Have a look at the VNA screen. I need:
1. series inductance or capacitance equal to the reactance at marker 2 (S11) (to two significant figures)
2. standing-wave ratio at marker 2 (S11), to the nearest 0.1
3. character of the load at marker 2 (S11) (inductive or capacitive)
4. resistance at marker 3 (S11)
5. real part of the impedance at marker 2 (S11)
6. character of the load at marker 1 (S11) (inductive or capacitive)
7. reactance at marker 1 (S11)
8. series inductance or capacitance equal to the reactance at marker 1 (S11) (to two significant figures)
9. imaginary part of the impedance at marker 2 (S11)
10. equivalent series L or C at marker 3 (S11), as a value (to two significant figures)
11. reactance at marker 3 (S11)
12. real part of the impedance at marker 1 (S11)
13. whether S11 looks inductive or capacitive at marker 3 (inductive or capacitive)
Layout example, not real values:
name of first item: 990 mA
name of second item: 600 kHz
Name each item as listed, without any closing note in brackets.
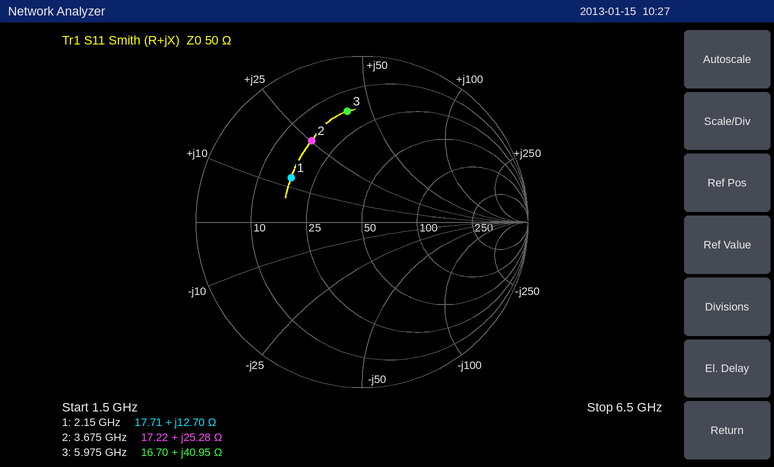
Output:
series inductance or capacitance equal to the reactance at marker 2 (S11): 1.1 nH
standing-wave ratio at marker 2 (S11), to the nearest 0.1: 3.7
character of the load at marker 2 (S11): inductive
resistance at marker 3: 16.70 Ω
real part of the impedance at marker 2: 17.22 Ω
character of the load at marker 1 (S11): inductive
reactance at marker 1: +12.70 Ω
series inductance or capacitance equal to the reactance at marker 1 (S11): 940 pH
imaginary part of the impedance at marker 2: +25.28 Ω
equivalent series L or C at marker 3 (S11), as a value: 1.1 nH
reactance at marker 3: +40.95 Ω
real part of the impedance at marker 1: 17.71 Ω
whether S11 looks inductive or capacitive at marker 3: inductive
